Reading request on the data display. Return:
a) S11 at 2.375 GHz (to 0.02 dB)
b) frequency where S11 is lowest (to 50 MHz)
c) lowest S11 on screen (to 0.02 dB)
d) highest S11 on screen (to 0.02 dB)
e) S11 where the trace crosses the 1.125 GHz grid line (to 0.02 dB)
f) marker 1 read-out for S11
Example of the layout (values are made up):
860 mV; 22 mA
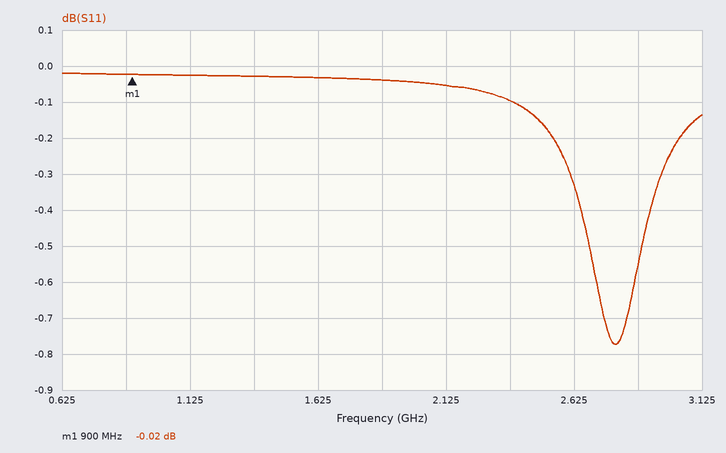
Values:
-0.10 dB; 2.80 GHz; -0.78 dB; -0.02 dB; -0.02 dB; -0.02 dB
